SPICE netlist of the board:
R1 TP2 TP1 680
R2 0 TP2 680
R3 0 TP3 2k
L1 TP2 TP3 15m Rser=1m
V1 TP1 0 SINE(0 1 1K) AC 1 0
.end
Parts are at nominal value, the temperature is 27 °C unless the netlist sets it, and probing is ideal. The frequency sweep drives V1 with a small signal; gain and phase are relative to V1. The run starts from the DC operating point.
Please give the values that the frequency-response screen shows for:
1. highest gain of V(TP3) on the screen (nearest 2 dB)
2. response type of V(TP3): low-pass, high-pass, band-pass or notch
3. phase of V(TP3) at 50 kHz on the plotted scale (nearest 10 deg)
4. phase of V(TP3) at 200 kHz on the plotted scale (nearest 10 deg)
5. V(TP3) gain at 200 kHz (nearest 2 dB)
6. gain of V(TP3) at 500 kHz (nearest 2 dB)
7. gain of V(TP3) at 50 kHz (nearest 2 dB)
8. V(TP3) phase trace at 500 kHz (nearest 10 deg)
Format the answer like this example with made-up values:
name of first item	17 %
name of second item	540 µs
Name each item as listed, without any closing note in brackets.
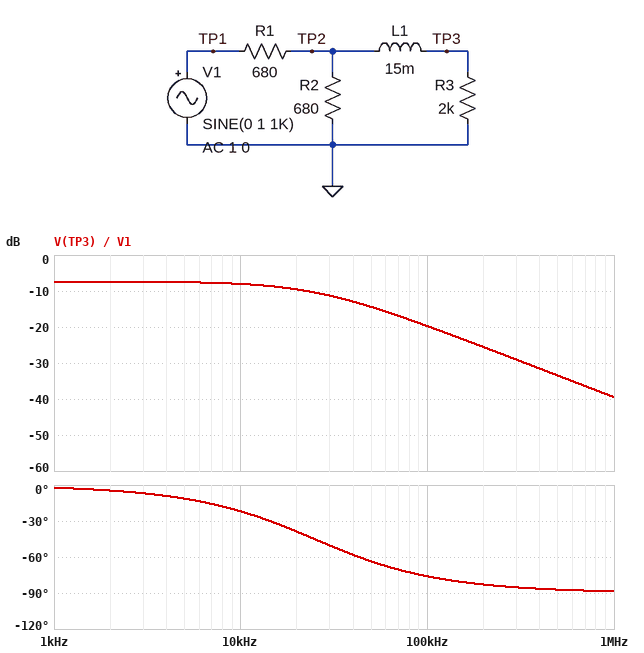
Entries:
highest gain of V(TP3) on the screen	-8 dB
response type of V(TP3): low-pass, high-pass, band-pass or notch	low-pass
phase of V(TP3) at 50 kHz on the plotted scale	-60 deg
phase of V(TP3) at 200 kHz on the plotted scale	-80 deg
V(TP3) gain at 200 kHz	-26 dB
gain of V(TP3) at 500 kHz	-34 dB
gain of V(TP3) at 50 kHz	-14 dB
V(TP3) phase trace at 500 kHz	-90 deg
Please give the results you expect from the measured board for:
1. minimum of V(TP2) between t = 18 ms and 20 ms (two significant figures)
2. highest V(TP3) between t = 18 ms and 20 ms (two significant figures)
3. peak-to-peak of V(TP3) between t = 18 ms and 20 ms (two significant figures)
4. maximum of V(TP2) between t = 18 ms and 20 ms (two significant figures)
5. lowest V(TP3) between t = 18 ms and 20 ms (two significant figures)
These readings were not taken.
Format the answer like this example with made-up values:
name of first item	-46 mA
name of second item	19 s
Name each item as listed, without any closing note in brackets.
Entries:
minimum of V(TP2) between t = 18 ms and 20 ms	-430 mV
highest V(TP3) between t = 18 ms and 20 ms	430 mV
peak-to-peak of V(TP3) between t = 18 ms and 20 ms	850 mV
maximum of V(TP2) between t = 18 ms and 20 ms	430 mV
lowest V(TP3) between t = 18 ms and 20 ms	-430 mV
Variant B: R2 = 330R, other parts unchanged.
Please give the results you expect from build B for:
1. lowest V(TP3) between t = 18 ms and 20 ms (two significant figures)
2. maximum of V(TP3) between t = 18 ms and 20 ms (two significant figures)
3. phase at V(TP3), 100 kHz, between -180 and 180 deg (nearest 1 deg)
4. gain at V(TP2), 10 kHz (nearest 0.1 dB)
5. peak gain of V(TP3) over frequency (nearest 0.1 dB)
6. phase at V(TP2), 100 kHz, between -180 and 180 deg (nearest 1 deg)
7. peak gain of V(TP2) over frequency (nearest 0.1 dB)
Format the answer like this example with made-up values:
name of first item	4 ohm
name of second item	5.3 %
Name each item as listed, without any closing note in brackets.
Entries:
lowest V(TP3) between t = 18 ms and 20 ms	-290 mV
maximum of V(TP3) between t = 18 ms and 20 ms	290 mV
phase at V(TP3), 100 kHz, between -180 and 180 deg	-77 deg
gain at V(TP2), 10 kHz	-10.5 dB
peak gain of V(TP3) over frequency	-10.6 dB
phase at V(TP2), 100 kHz, between -180 and 180 deg	1 deg
peak gain of V(TP2) over frequency	-9.7 dB
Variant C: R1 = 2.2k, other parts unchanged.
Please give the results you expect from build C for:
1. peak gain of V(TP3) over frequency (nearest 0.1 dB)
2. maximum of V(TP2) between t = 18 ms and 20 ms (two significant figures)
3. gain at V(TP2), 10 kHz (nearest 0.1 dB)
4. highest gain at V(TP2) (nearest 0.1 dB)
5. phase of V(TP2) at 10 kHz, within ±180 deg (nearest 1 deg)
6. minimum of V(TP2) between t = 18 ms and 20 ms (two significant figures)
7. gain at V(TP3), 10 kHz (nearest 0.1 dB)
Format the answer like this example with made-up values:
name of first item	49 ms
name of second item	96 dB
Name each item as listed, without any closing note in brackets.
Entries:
peak gain of V(TP3) over frequency	-14.5 dB
maximum of V(TP2) between t = 18 ms and 20 ms	190 mV
gain at V(TP2), 10 kHz	-14.2 dB
highest gain at V(TP2)	-12.5 dB
phase of V(TP2) at 10 kHz, within ±180 deg	5 deg
minimum of V(TP2) between t = 18 ms and 20 ms	-190 mV
gain at V(TP3), 10 kHz	-15.1 dB
